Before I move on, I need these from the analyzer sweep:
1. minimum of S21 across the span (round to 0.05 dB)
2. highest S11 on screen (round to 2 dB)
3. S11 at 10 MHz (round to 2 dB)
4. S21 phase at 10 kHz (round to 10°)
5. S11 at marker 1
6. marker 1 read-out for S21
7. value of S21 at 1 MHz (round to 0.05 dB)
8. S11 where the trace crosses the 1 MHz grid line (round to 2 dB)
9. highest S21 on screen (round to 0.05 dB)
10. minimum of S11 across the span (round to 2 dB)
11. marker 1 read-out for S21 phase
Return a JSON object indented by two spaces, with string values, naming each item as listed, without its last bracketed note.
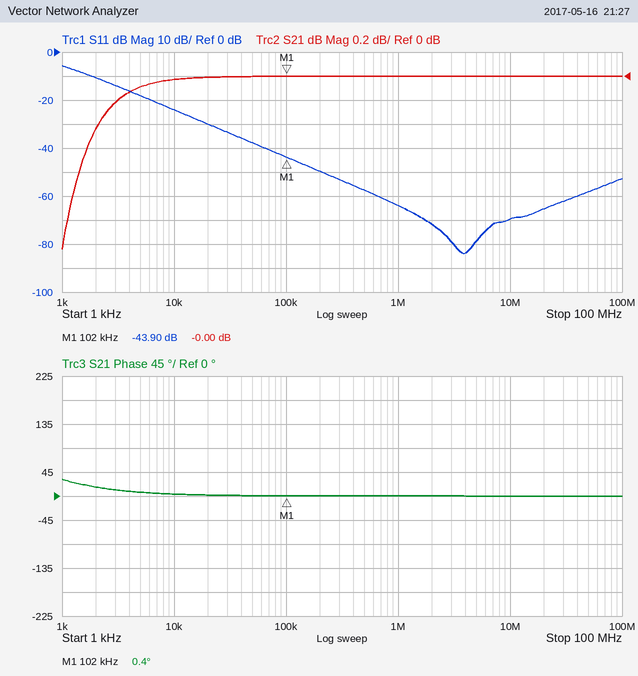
{
  "minimum of S21 across the span": "-1.45 dB",
  "highest S11 on screen": "-6 dB",
  "S11 at 10 MHz": "-70 dB",
  "S21 phase at 10 kHz": "0°",
  "S11 at marker 1": "-43.90 dB",
  "marker 1 read-out for S21": "-0.00 dB",
  "value of S21 at 1 MHz": "0.00 dB",
  "S11 where the trace crosses the 1 MHz grid line": "-64 dB",
  "highest S21 on screen": "0.00 dB",
  "minimum of S11 across the span": "-84 dB",
  "marker 1 read-out for S21 phase": "0.4°"
}
